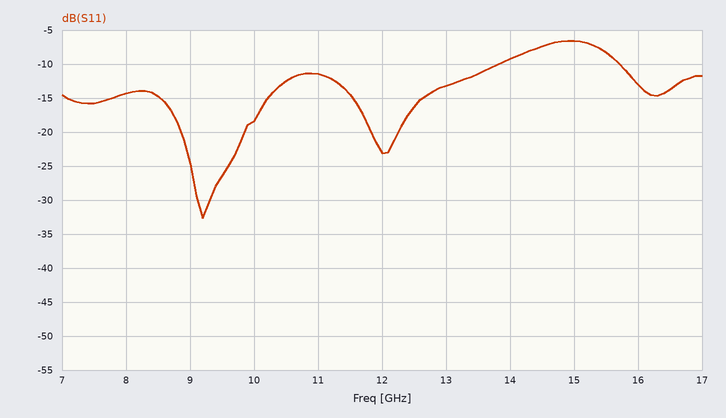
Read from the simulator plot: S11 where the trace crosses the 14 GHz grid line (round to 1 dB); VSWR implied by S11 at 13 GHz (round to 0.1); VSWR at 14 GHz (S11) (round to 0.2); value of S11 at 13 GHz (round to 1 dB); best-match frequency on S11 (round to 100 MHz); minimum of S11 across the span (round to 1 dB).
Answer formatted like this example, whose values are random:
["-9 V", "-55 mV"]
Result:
["-9 dB", "1.6", "2.0", "-13 dB", "9.2 GHz", "-33 dB"]
